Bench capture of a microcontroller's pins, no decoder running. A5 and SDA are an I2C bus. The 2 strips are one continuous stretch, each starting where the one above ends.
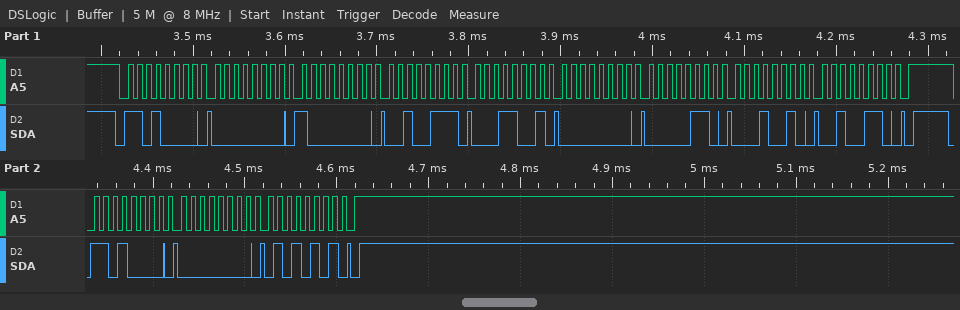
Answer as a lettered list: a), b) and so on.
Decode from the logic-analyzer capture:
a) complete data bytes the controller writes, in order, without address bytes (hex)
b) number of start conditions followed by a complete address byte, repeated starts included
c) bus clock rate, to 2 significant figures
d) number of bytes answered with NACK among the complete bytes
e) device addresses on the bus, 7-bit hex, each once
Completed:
a) 00 80 27 19 00 06 12 26 00 55
b) 2
c) 100 kHz
d) 0
e) 0x68
